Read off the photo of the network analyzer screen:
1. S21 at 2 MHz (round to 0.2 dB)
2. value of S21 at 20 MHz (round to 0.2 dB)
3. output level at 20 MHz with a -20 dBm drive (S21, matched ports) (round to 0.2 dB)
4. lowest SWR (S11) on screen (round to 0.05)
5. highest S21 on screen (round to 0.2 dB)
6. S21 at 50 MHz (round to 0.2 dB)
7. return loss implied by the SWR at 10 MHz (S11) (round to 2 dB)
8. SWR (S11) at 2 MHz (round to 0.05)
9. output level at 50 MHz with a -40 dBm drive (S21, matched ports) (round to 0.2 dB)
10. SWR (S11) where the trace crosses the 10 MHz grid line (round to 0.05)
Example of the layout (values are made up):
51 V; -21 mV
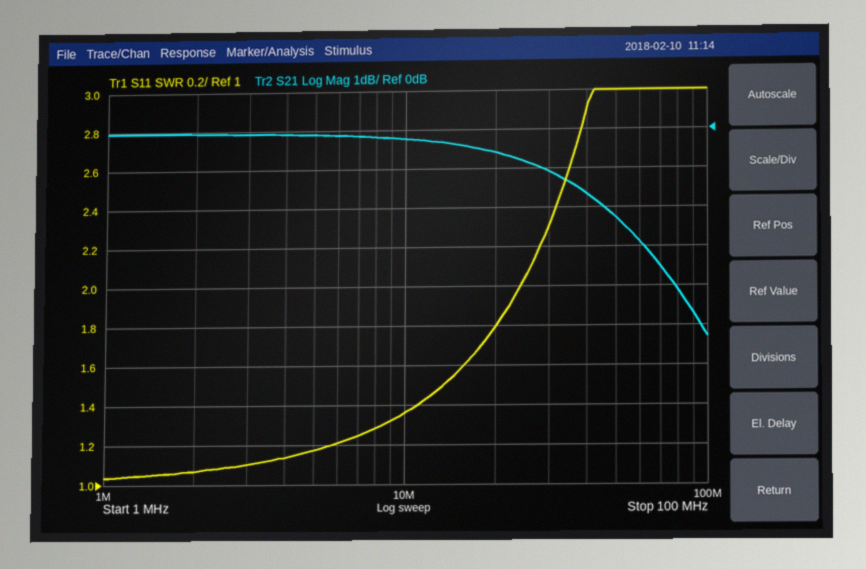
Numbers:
0.0 dB; -0.6 dB; -20.6 dBm; 1.05; 0.0 dB; -2.2 dB; 16 dB; 1.05; -42.2 dBm; 1.35
